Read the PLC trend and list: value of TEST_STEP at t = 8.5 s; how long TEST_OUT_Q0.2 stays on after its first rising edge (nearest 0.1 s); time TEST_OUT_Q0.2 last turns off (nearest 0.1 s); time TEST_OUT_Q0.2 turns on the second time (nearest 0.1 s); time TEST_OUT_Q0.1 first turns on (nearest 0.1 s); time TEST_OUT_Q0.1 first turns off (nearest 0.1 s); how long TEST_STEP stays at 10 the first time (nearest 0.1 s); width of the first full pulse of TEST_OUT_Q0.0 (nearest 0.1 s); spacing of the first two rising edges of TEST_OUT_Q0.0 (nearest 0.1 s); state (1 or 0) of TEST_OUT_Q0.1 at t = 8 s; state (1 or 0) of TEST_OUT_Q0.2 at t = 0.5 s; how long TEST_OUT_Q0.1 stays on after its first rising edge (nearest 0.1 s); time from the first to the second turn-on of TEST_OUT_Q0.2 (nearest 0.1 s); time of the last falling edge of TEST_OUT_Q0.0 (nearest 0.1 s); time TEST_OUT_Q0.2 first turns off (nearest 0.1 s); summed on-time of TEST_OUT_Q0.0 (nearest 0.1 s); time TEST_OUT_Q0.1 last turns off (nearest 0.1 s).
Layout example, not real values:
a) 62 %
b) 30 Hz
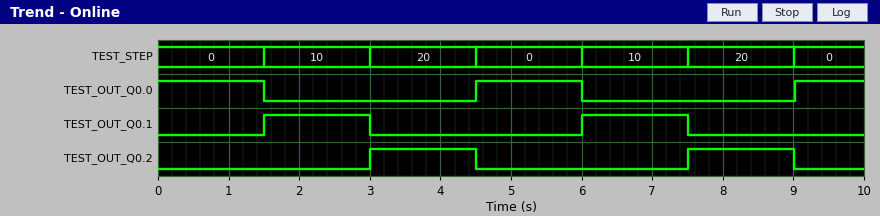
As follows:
a) 20
b) 1.5 s
c) 9.0 s
d) 7.5 s
e) 1.5 s
f) 3.0 s
g) 1.5 s
h) 1.5 s
i) 4.5 s
j) 0
k) 0
l) 1.5 s
m) 4.5 s
n) 6.0 s
o) 4.5 s
p) 4.0 s
q) 7.5 s
